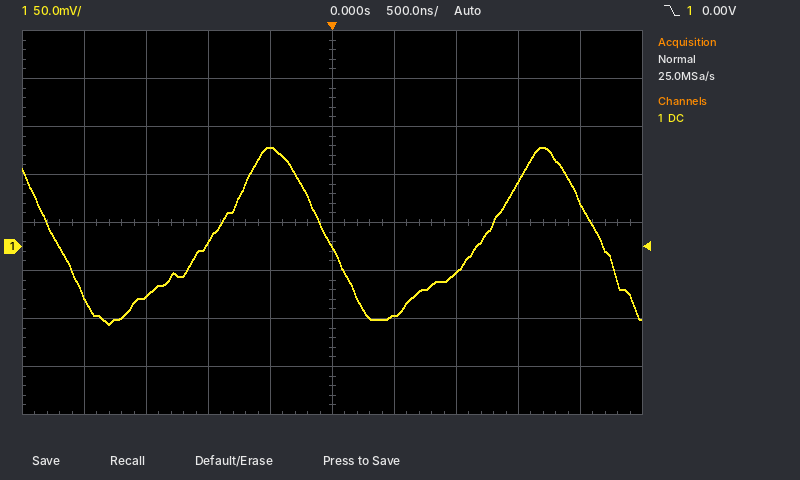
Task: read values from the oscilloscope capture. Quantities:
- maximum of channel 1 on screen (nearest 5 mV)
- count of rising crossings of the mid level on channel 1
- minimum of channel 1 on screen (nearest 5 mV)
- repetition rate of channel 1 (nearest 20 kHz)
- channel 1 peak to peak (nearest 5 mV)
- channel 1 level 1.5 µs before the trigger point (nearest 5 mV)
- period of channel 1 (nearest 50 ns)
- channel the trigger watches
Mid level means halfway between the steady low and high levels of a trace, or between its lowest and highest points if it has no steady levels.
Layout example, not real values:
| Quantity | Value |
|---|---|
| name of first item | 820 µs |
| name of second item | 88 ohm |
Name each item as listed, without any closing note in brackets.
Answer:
| Quantity | Value |
|---|---|
| maximum of channel 1 on screen | 105 mV |
| count of rising crossings of the mid level on channel 1 | 2 |
| minimum of channel 1 on screen | -80 mV |
| repetition rate of channel 1 | 460 kHz |
| channel 1 peak to peak | 185 mV |
| channel 1 level 1.5 µs before the trigger point | -50 mV |
| period of channel 1 | 2.20 µs |
| channel the trigger watches | channel 1 |
